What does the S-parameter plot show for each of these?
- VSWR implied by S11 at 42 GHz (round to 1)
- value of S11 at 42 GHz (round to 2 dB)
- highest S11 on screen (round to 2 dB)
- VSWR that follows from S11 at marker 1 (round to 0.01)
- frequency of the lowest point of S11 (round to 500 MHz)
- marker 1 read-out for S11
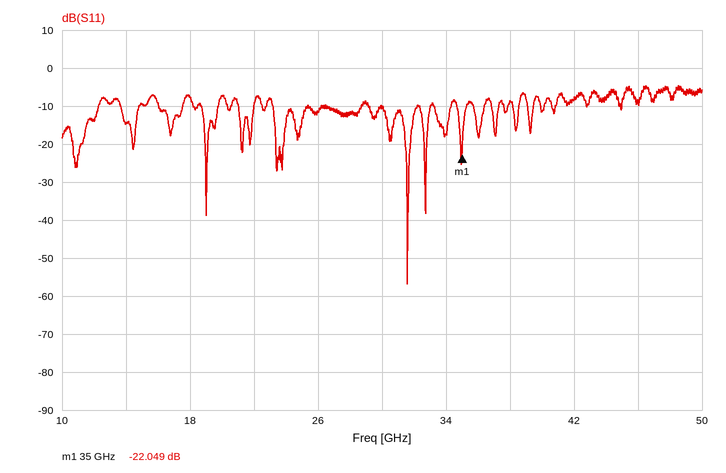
2
-8 dB
-4 dB
1.17
31.5 GHz
-22.049 dB
